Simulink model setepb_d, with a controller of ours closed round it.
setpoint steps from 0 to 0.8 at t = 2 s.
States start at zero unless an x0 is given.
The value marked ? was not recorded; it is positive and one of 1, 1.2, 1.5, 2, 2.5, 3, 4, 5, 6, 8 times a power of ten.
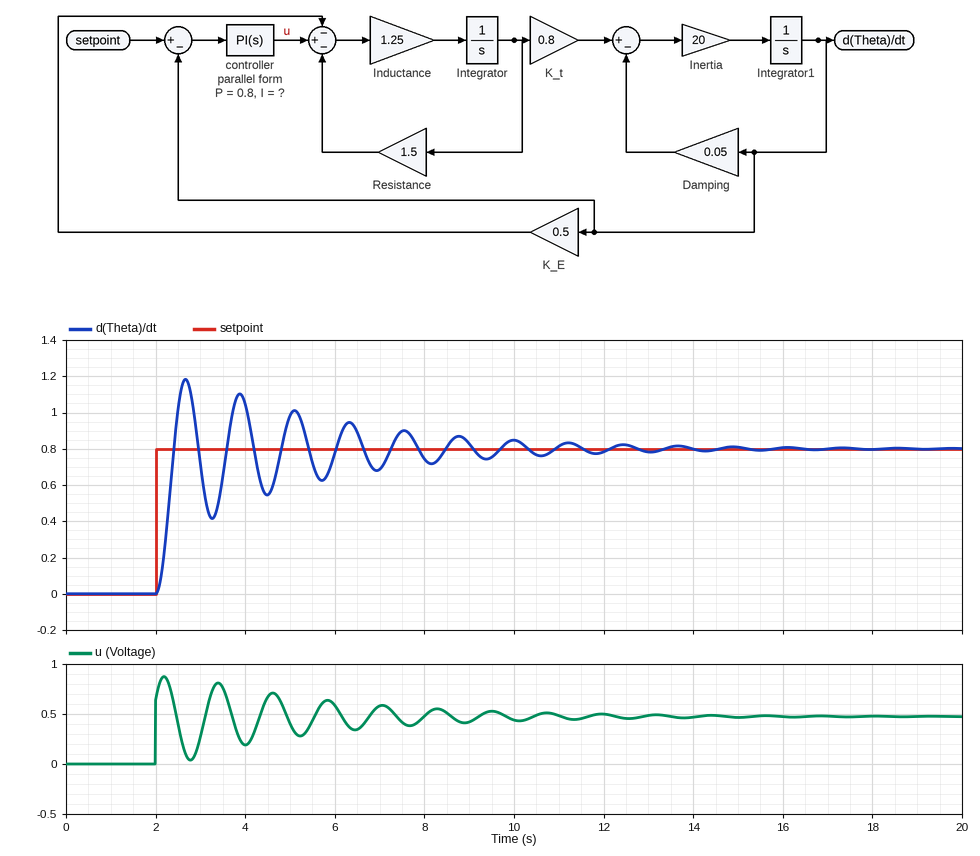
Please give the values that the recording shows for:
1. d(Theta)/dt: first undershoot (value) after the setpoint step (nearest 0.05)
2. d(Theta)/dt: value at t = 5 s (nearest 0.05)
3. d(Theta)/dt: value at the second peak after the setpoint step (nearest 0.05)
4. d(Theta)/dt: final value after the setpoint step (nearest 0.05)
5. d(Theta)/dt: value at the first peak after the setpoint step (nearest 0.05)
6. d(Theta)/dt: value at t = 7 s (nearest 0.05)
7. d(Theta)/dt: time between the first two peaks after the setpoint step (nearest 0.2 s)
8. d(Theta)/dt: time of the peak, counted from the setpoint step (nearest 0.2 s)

0.40
1.00
1.10
0.80
1.20
0.70
1.2 s
0.6 s
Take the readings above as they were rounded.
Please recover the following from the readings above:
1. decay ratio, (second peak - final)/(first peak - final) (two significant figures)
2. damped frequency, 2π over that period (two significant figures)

0.75
5.2 rad/s
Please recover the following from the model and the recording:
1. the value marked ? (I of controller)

3
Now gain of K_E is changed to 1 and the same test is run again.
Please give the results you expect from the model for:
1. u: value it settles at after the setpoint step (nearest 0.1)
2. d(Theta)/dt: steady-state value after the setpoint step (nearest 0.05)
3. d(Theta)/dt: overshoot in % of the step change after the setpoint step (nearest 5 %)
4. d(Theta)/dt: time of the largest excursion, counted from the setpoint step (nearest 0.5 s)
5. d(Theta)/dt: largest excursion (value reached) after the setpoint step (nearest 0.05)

0.9
0.80
15 %
1.5 s
0.90
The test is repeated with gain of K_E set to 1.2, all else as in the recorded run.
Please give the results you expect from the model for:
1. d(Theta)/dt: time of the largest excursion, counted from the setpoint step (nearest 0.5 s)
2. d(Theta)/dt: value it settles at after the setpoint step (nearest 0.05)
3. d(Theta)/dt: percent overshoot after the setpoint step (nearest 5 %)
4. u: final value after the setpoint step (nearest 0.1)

1.5 s
0.80
10 %
1.0
